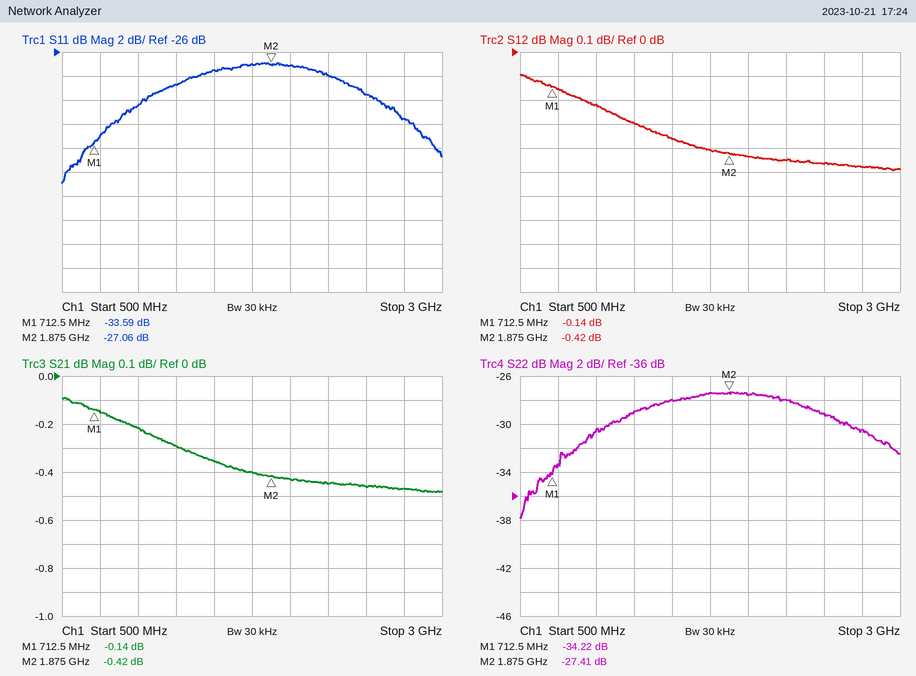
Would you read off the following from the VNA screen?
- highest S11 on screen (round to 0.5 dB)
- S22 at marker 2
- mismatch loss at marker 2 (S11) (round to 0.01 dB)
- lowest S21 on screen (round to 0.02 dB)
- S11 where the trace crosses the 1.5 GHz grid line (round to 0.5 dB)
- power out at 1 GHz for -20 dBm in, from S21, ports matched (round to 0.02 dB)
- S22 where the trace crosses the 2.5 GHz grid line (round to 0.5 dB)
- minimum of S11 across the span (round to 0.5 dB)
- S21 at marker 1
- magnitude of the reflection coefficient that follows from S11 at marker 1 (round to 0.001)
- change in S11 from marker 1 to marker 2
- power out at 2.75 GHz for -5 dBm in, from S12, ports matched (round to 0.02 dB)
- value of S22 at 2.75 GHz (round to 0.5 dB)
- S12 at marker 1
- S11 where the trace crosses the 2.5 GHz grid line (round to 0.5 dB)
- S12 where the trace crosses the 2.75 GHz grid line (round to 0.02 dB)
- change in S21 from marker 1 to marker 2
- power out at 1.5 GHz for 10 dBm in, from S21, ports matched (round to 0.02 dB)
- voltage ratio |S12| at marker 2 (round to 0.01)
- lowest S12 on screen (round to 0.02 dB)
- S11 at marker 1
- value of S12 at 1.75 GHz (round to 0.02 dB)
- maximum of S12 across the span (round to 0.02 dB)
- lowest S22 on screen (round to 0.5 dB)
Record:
-27.0 dB
-27.41 dB
0.01 dB
-0.48 dB
-27.5 dB
-20.22 dBm
-29.0 dB
-37.0 dB
-0.14 dB
0.021
6.53 dB
-5.48 dBm
-30.5 dB
-0.14 dB
-29.5 dB
-0.48 dB
-0.28 dB
9.64 dBm
0.95
-0.50 dB
-33.59 dB
-0.40 dB
-0.10 dB
-38.0 dB
